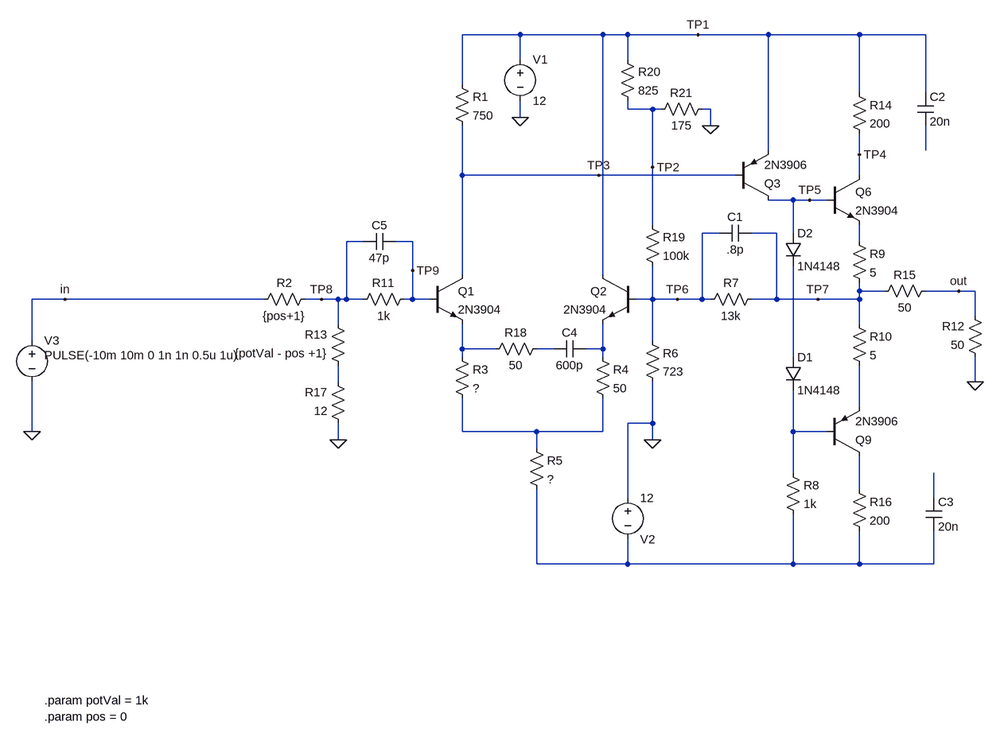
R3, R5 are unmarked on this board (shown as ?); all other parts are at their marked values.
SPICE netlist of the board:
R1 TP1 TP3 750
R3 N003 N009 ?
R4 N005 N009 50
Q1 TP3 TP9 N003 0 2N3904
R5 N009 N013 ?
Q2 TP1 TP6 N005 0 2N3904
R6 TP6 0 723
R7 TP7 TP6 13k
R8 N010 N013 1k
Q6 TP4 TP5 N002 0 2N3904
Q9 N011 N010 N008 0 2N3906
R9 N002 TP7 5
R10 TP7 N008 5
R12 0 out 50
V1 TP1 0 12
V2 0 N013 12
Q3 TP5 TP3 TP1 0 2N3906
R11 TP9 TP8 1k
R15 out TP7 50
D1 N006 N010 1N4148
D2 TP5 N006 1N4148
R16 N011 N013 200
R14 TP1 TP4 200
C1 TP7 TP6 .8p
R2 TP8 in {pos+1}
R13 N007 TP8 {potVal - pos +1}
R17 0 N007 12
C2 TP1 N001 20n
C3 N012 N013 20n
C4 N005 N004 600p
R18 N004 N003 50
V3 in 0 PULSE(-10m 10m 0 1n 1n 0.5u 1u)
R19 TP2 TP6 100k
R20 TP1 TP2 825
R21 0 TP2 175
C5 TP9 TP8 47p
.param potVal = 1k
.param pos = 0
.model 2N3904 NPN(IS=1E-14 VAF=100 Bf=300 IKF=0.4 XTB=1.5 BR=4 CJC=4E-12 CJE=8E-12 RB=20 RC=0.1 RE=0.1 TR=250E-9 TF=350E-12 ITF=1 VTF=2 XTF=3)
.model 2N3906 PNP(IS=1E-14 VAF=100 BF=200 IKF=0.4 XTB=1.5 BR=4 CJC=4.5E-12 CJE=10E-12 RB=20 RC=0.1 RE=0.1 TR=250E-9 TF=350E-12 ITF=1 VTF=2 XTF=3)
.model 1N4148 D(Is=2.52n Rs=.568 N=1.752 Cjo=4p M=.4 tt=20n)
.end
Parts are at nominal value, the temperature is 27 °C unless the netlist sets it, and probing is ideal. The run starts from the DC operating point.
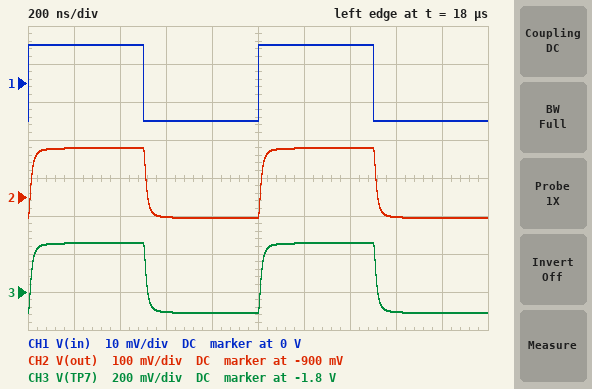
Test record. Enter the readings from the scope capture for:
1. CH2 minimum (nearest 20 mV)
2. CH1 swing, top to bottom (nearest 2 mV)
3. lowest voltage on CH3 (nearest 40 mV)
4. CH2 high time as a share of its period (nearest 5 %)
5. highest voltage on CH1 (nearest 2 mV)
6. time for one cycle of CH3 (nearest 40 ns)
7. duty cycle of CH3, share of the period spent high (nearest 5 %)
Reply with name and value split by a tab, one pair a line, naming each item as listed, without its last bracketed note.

CH2 minimum	-960 mV
CH1 swing, top to bottom	20 mV
lowest voltage on CH3	-1.92 V
CH2 high time as a share of its period	50 %
highest voltage on CH1	10 mV
time for one cycle of CH3	1.00 µs
duty cycle of CH3, share of the period spent high	50 %
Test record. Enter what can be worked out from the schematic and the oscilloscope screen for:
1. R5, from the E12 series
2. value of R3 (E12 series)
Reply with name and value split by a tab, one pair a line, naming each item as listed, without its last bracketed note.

R5, from the E12 series	8.2 kΩ
value of R3	68 Ω
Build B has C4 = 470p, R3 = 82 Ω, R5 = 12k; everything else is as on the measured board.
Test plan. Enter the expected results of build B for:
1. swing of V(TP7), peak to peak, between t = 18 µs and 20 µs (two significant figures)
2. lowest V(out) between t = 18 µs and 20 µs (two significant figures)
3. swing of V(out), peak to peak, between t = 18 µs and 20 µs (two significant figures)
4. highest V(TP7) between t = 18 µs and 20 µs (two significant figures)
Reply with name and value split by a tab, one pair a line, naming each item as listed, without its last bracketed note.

swing of V(TP7), peak to peak, between t = 18 µs and 20 µs	31 mV
lowest V(out) between t = 18 µs and 20 µs	-2.1 V
swing of V(out), peak to peak, between t = 18 µs and 20 µs	15 mV
highest V(TP7) between t = 18 µs and 20 µs	-4.1 V
